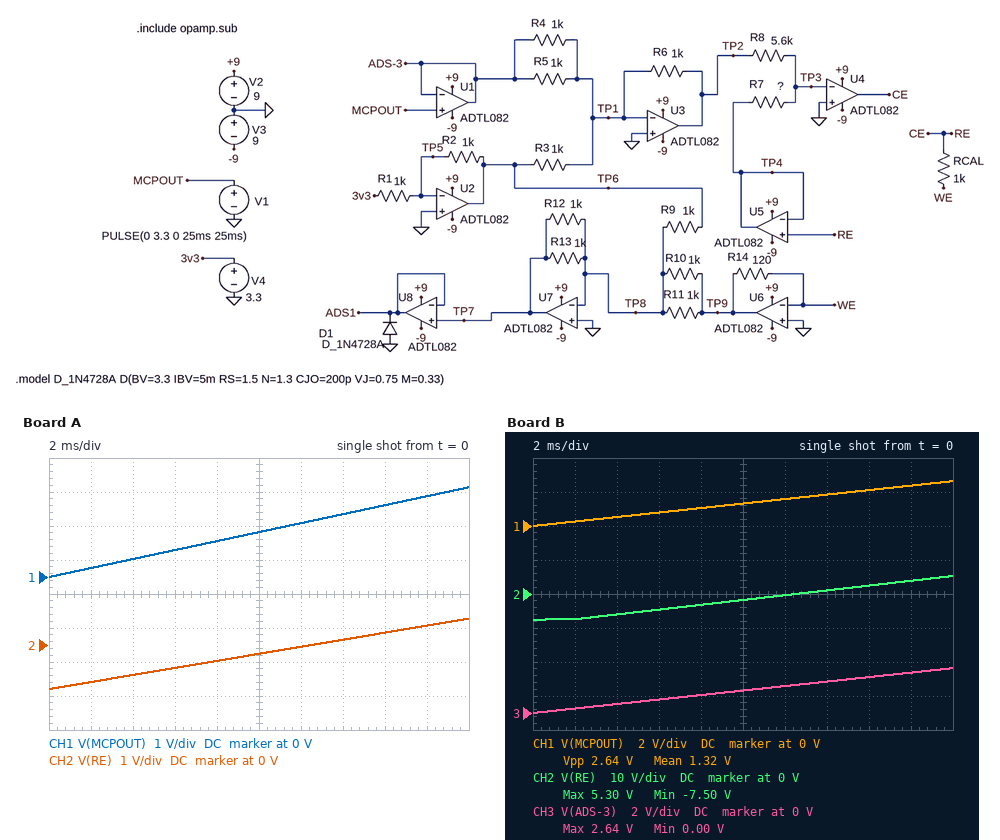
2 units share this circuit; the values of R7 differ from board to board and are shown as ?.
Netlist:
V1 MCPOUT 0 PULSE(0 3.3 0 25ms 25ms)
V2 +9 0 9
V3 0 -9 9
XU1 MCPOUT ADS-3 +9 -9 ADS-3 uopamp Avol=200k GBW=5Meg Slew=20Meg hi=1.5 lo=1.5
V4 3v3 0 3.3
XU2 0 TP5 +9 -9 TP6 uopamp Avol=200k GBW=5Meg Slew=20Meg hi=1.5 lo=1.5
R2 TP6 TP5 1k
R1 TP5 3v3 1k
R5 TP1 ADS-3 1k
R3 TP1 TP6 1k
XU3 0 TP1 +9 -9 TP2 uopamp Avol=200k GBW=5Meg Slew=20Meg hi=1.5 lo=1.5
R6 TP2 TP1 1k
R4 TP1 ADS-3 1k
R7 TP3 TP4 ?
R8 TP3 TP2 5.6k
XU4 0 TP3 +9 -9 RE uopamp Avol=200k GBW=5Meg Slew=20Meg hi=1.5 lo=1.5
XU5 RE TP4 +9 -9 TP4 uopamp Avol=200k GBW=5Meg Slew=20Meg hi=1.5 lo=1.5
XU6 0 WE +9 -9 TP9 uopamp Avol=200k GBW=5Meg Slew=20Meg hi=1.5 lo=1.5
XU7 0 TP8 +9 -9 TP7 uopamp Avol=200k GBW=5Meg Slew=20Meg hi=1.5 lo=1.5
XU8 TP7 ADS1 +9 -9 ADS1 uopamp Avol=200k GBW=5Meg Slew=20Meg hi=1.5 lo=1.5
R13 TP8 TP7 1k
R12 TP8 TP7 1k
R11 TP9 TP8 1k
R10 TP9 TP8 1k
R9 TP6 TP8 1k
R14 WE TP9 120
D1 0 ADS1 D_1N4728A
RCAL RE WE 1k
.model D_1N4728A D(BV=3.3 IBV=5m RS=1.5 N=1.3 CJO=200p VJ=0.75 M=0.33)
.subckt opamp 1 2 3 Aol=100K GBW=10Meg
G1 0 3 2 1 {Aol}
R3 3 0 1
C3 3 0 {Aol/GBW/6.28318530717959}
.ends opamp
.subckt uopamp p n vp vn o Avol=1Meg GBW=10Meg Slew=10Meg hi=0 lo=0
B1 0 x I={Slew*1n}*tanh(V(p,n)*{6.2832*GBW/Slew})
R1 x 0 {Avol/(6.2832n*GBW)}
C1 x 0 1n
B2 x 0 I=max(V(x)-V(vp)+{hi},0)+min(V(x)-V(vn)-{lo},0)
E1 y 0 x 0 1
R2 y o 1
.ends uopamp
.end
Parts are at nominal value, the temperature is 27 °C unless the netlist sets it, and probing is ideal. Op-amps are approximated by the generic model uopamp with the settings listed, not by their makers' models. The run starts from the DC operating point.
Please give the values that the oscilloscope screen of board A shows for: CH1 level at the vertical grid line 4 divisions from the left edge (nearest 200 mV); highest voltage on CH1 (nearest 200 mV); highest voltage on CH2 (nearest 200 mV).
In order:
1.0 V
2.6 V
800 mV
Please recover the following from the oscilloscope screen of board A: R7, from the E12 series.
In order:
2.2 kΩ
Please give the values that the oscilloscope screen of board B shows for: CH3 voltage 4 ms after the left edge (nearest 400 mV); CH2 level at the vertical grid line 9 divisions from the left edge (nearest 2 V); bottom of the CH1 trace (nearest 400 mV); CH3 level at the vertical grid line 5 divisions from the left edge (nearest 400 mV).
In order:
400 mV
4 V
0 V
1.2 V
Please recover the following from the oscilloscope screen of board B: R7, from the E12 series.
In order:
15 kΩ
